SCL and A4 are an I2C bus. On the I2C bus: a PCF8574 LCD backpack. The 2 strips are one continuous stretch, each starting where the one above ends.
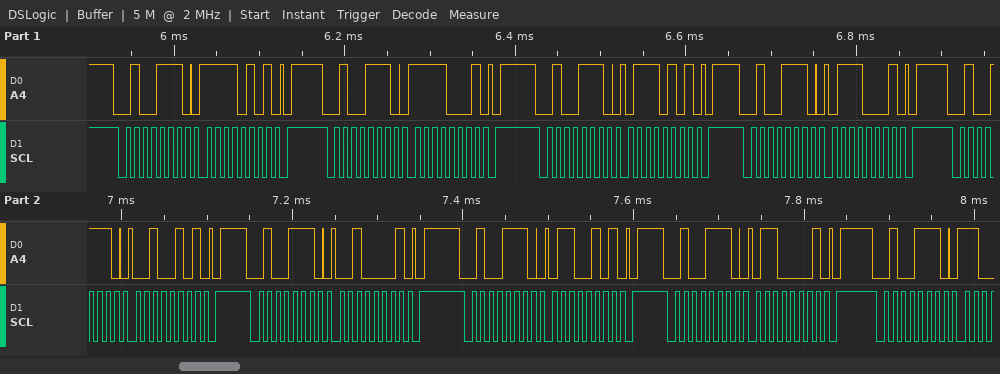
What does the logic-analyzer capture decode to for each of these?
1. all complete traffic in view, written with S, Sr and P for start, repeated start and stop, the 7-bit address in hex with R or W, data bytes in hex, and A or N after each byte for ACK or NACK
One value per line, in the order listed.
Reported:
S 27W A F5 A P S 27W A F1 A P S 27W A 75 A P S 27W A 71 A P S 27W A 25 A P S 27W A 21 A P S 27W A 65 A P S 27W A 61 A P S 27W A
